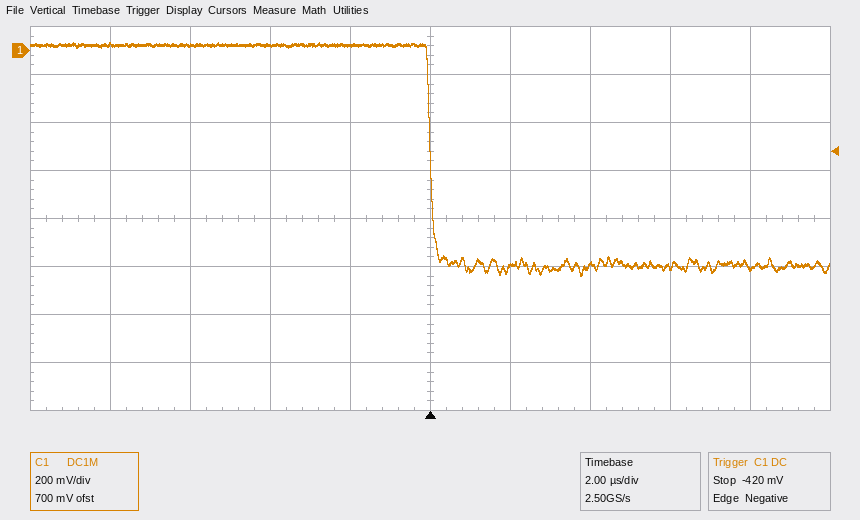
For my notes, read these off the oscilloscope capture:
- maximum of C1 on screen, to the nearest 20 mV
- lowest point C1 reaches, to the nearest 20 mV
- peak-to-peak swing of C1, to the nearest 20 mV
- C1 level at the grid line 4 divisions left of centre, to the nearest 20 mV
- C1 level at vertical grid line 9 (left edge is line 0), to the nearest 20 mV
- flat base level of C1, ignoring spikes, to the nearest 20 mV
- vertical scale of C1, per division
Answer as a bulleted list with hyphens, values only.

- 40 mV
- -940 mV
- 980 mV
- 20 mV
- -900 mV
- -900 mV
- 200 mV
